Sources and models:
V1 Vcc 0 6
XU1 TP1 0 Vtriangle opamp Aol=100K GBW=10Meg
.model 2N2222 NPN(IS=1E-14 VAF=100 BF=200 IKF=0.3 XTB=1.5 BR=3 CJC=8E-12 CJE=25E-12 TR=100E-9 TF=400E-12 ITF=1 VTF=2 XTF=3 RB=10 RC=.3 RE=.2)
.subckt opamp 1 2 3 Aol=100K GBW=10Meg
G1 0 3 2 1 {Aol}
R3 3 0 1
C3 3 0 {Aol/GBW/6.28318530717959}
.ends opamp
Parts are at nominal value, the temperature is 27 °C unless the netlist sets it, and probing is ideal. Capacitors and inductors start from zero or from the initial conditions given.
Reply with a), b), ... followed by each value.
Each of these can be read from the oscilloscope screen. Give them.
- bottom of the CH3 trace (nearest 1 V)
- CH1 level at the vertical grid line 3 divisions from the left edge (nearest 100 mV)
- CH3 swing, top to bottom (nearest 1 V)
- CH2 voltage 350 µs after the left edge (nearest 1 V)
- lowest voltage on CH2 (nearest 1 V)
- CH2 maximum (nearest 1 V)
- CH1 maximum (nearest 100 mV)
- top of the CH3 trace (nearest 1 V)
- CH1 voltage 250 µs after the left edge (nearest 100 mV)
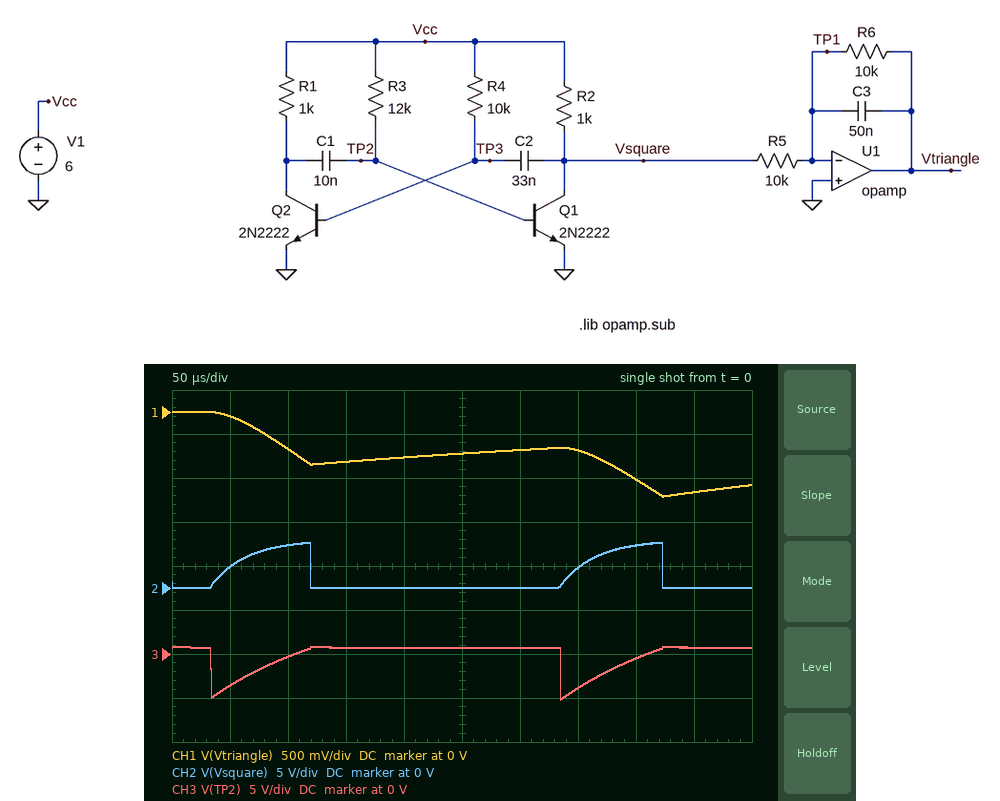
a) -5 V
b) -600 mV
c) 6 V
d) 2 V
e) 0 V
f) 5 V
g) 0 V
h) 1 V
i) -500 mV
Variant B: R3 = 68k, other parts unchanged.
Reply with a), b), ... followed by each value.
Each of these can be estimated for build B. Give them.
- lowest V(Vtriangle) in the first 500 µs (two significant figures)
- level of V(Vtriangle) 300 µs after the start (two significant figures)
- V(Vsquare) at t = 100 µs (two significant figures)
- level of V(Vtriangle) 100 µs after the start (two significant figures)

a) -3.2 V
b) -2.1 V
c) 4.9 V
d) -440 mV
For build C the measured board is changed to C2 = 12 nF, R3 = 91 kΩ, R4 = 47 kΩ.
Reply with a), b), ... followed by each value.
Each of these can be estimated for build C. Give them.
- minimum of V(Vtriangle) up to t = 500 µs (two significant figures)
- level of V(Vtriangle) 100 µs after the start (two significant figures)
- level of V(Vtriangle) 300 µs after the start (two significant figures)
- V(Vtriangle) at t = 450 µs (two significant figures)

a) -750 mV
b) -660 mV
c) -480 mV
d) -380 mV
